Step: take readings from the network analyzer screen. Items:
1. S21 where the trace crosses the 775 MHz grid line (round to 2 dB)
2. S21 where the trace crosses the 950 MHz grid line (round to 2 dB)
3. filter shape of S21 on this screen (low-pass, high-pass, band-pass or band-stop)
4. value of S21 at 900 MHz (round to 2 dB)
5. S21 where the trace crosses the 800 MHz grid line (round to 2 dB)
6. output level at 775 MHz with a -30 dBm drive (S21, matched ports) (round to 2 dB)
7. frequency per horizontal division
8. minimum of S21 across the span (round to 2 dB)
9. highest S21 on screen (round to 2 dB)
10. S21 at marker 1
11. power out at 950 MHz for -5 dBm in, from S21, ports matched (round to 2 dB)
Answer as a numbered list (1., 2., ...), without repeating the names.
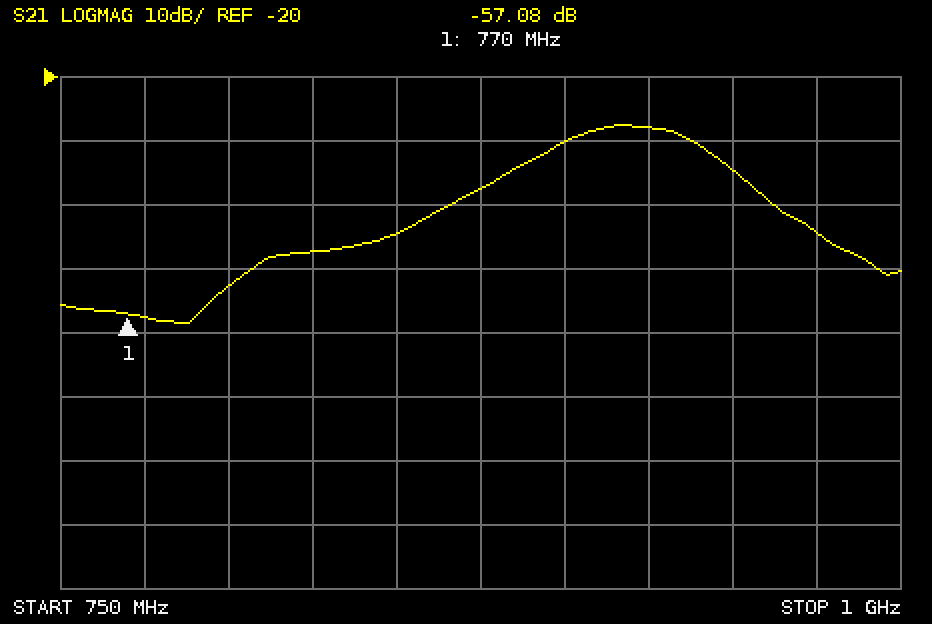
1. -58 dB
2. -34 dB
3. band-pass
4. -30 dB
5. -52 dB
6. -88 dBm
7. 25 MHz
8. -58 dB
9. -28 dB
10. -57.08 dB
11. -40 dBm
